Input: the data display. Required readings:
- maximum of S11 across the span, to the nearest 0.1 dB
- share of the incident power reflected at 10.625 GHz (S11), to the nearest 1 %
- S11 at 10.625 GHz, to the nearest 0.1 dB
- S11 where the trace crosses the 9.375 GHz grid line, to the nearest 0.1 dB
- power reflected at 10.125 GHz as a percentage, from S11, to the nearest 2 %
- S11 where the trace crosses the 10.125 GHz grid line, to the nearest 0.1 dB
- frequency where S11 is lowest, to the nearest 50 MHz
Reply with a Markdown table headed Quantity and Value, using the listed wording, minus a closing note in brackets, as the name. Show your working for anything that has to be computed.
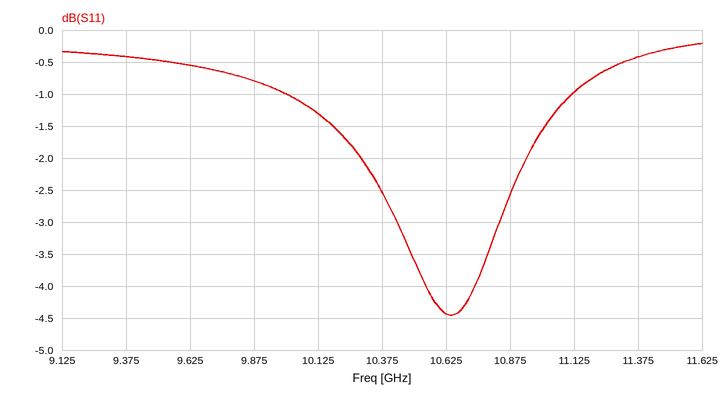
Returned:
| Quantity | Value |
|---|---|
| maximum of S11 across the span, to the nearest 0.1 dB | -0.2 dB |
| share of the incident power reflected at 10.625 GHz (S11), to the nearest 1 % | 10^(-4.4/10) ≈ 36 % |
| S11 at 10.625 GHz, to the nearest 0.1 dB | -4.4 dB |
| S11 where the trace crosses the 9.375 GHz grid line, to the nearest 0.1 dB | -0.4 dB |
| power reflected at 10.125 GHz as a percentage, from S11, to the nearest 2 % | 10^(-1.3/10) ≈ 74 % |
| S11 where the trace crosses the 10.125 GHz grid line, to the nearest 0.1 dB | -1.3 dB |
| frequency where S11 is lowest, to the nearest 50 MHz | 10.65 GHz |
